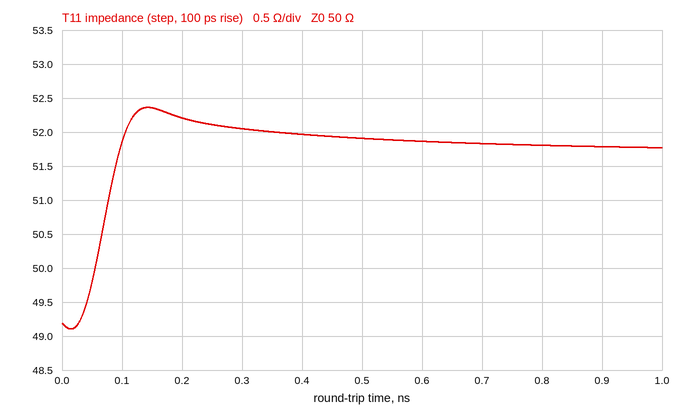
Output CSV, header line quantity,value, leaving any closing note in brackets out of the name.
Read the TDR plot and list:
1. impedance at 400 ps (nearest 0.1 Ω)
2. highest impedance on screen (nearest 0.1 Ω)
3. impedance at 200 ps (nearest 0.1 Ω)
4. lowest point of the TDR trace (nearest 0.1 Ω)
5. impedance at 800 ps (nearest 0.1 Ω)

quantity,value
impedance at 400 ps,52.0 Ω
highest impedance on screen,52.4 Ω
impedance at 200 ps,52.2 Ω
lowest point of the TDR trace,49.1 Ω
impedance at 800 ps,51.8 Ω
